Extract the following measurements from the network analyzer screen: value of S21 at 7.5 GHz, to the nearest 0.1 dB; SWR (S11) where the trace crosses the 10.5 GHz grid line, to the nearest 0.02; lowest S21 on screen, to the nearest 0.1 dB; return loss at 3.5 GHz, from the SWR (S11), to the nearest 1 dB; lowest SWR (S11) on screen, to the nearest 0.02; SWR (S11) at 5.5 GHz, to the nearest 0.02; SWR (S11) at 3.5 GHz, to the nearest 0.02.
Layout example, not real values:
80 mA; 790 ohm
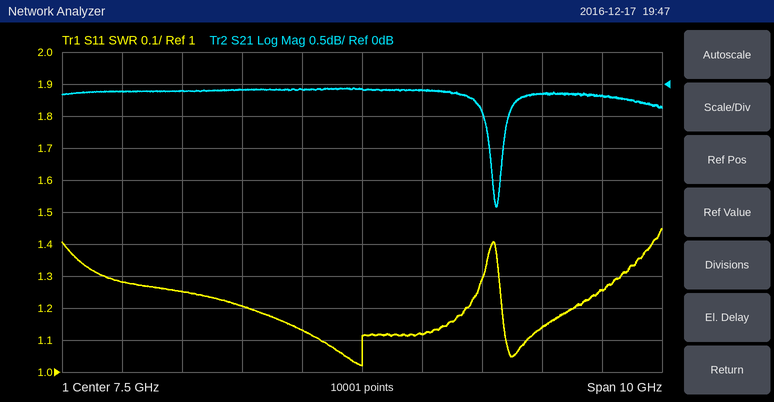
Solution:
-0.1 dB; 1.14; -1.9 dB; 18 dB; 1.02; 1.20; 1.28
